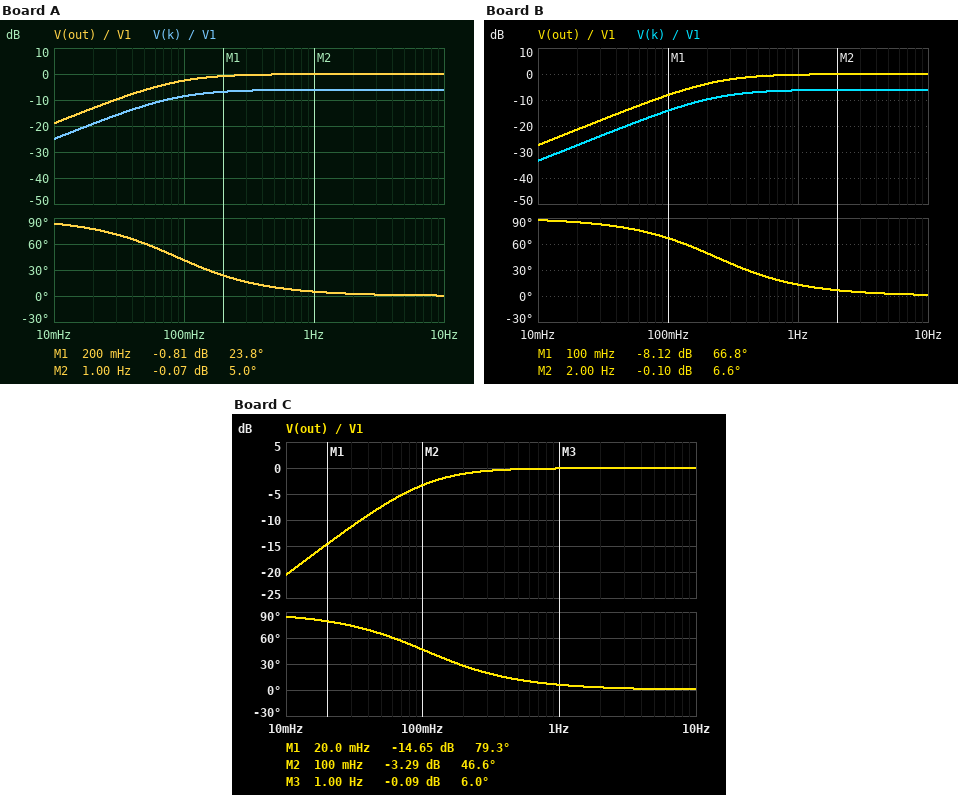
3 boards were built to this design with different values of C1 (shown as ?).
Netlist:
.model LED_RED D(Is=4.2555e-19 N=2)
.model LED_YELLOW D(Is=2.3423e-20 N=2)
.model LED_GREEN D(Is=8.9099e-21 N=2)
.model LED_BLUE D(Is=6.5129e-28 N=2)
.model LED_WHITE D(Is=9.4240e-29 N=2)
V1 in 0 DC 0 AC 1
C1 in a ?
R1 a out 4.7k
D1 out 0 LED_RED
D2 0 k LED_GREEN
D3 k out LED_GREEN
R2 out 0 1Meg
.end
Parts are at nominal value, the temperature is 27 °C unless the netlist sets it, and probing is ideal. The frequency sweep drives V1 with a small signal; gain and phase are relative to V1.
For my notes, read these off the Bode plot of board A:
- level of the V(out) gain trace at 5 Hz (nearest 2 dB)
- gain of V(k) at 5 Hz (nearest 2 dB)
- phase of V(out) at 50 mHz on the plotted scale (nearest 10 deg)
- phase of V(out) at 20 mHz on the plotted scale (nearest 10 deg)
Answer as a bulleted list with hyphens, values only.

- 0 dB
- -6 dB
- 60 deg
- 80 deg
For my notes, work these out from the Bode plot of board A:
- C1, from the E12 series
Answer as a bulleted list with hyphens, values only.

- 1.8 µF
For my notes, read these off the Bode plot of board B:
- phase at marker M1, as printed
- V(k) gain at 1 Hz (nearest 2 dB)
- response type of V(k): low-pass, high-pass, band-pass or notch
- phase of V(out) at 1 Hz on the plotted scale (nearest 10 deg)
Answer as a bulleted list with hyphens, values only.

- 66.8 deg
- -6 dB
- high-pass
- 10 deg
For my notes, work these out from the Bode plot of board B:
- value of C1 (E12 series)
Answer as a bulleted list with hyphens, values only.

- 680 nF
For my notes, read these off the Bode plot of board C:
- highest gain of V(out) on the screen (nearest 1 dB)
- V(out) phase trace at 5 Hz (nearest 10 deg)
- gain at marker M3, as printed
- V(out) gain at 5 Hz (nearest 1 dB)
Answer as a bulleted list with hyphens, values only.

- 0 dB
- 0 deg
- -0.09 dB
- 0 dB
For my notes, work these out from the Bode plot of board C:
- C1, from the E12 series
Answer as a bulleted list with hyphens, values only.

- 1.5 µF
